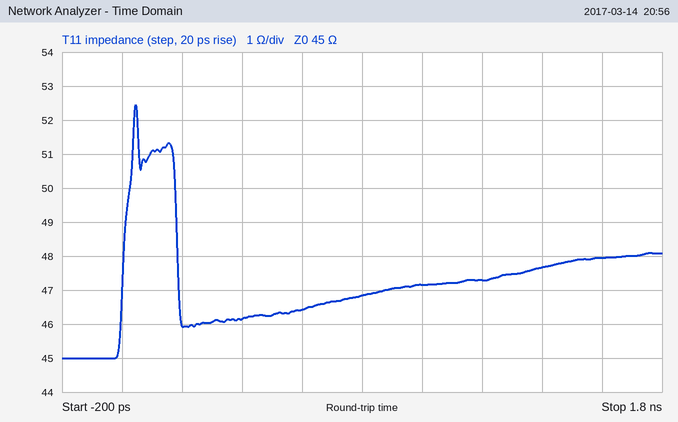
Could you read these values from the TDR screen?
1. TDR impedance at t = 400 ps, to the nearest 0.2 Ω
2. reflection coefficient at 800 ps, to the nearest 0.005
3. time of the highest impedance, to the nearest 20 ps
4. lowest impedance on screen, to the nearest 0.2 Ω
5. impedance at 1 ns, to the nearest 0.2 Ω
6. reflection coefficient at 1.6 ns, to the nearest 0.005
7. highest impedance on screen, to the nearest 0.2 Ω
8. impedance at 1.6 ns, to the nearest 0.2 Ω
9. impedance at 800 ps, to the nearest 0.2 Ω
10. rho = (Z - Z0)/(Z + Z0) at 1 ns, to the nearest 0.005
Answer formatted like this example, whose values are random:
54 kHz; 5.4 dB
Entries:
46.2 Ω; +0.020; 40 ps; 45.0 Ω; 47.2 Ω; +0.030; 52.4 Ω; 48.0 Ω; 46.8 Ω; +0.025
